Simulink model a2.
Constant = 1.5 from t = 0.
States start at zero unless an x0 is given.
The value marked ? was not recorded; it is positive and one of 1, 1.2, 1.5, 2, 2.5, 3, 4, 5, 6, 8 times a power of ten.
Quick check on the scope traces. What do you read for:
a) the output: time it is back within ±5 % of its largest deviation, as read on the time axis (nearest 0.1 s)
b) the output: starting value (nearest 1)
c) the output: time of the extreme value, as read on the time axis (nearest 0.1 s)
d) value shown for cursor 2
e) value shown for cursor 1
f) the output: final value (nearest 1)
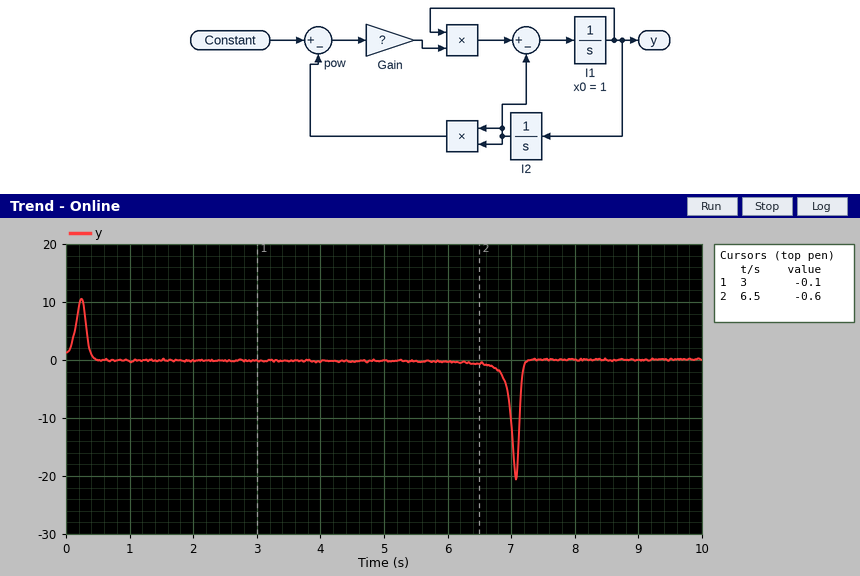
7.2 s
1
7.1 s
-0.6
-0.1
0
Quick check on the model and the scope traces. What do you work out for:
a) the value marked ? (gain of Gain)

8
